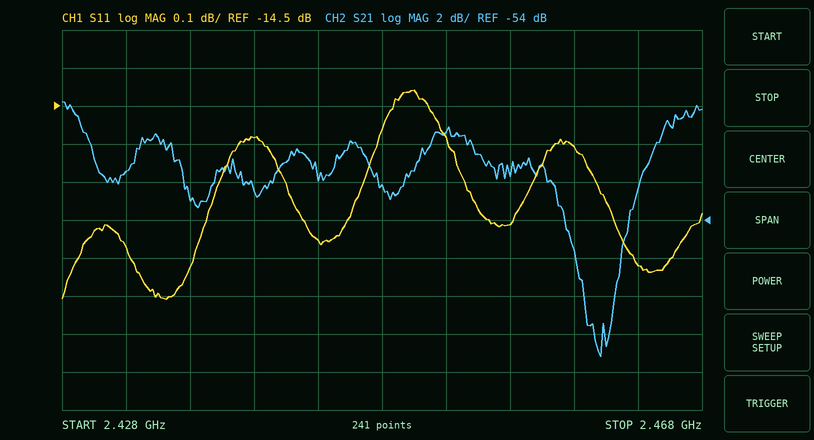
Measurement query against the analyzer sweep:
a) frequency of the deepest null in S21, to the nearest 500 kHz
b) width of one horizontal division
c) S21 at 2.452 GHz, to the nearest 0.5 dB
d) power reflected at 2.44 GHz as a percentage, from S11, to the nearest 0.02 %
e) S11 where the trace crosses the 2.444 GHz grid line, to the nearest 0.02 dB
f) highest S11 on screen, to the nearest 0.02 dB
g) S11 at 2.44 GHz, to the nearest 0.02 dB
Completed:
2.4615 GHz
4 MHz
-49.5 dB
3.48 %
-14.86 dB
-14.46 dB
-14.58 dB
